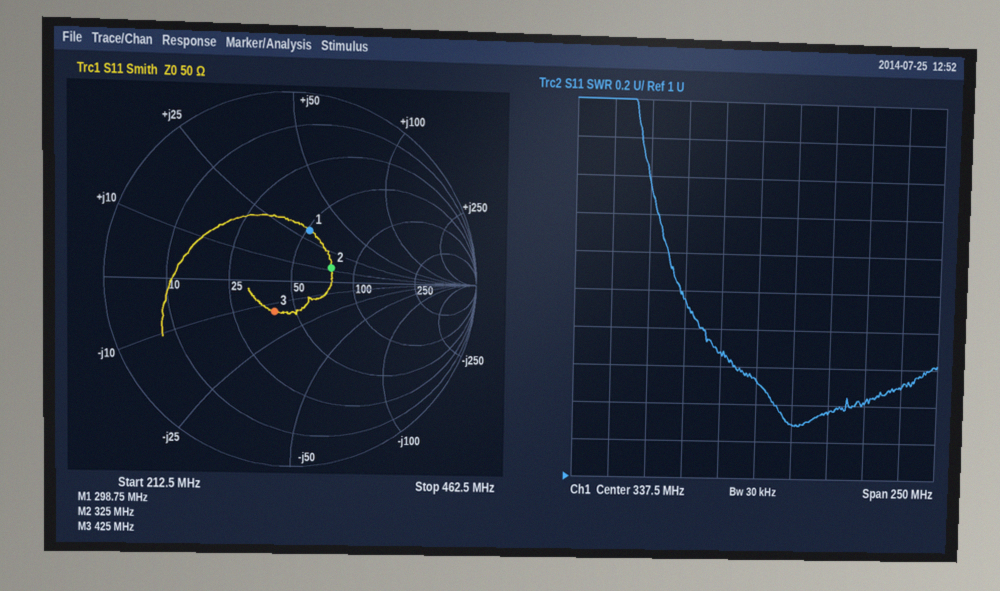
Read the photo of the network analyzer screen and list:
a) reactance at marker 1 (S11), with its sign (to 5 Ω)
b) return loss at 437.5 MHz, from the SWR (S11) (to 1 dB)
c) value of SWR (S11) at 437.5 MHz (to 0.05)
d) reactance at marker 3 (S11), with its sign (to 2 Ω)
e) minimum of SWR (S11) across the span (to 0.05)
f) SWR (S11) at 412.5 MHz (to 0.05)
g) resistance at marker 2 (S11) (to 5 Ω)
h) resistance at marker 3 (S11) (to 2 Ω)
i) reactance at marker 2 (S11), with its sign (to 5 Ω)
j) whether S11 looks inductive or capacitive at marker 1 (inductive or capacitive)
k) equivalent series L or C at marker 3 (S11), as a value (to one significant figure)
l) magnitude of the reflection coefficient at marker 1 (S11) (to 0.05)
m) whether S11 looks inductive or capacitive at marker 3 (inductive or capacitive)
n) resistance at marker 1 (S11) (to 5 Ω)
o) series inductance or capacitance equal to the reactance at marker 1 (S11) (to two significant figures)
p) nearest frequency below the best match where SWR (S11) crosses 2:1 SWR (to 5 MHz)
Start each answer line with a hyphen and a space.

- +30 Ω
- 14 dB
- 1.50
- -14 Ω
- 1.30
- 1.40
- 75 Ω
- 40 Ω
- +10 Ω
- inductive
- 30 pF
- 0.30
- capacitive
- 50 Ω
- 16 nH
- 285 MHz
